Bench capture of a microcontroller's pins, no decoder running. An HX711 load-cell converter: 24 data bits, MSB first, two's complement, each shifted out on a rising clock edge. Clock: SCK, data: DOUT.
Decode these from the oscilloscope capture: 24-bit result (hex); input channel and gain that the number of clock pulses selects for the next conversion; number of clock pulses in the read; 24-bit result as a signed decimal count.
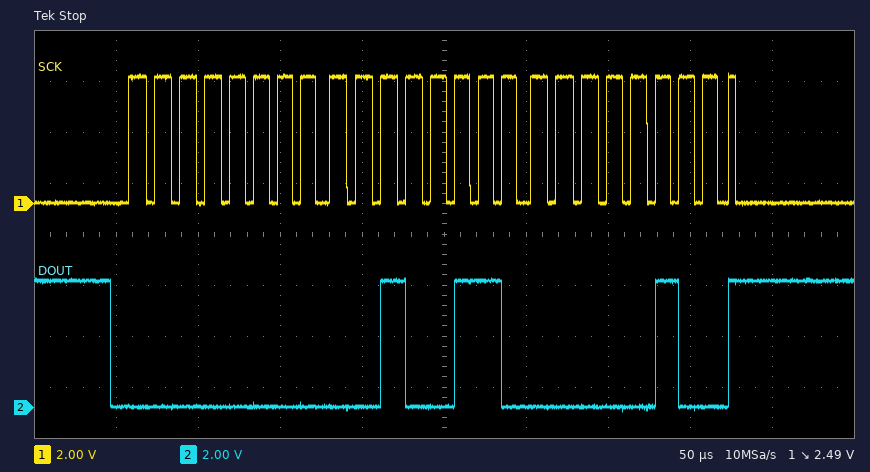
0x002604
channel A, gain 128
25
9732
